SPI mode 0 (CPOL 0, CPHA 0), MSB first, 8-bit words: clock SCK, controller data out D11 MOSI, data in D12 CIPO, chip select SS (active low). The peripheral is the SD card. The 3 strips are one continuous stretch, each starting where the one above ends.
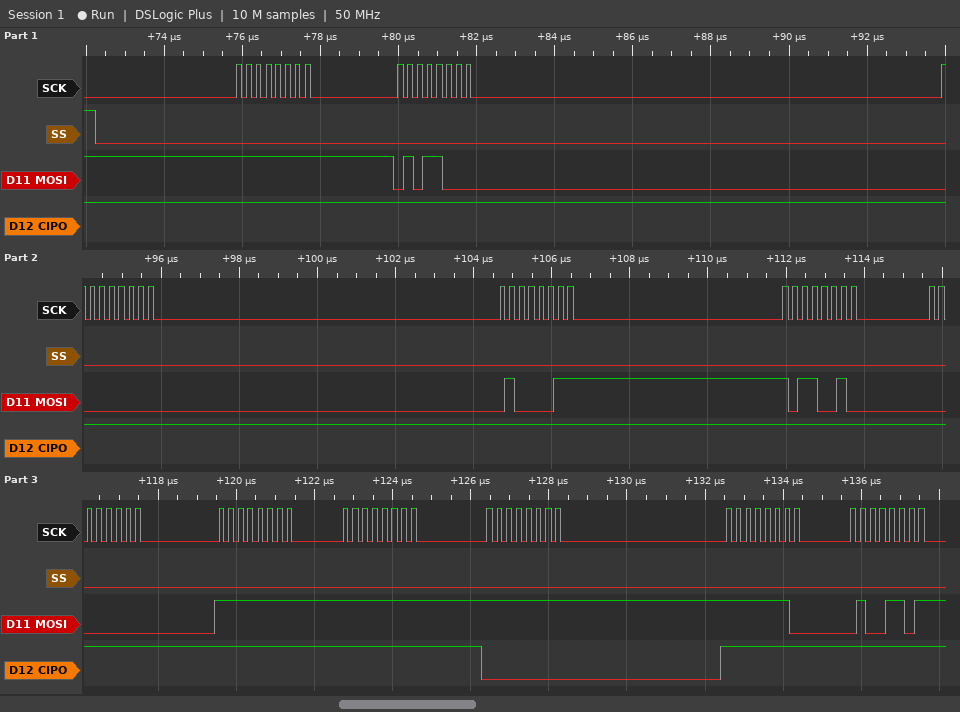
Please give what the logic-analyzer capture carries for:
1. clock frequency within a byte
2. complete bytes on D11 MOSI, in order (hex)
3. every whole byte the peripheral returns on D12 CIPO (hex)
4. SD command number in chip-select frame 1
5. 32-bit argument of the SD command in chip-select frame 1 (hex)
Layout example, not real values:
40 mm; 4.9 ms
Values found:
4 MHz; FF 58 00 43 B2 00 FF FF FF FE 4D; FF FF FF FF FF FF FF FF 00 FF FF; CMD24; 0x0043B200
